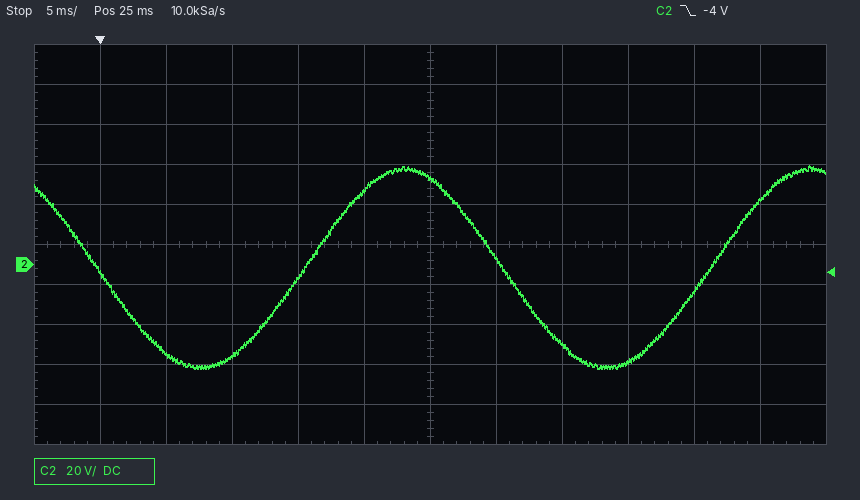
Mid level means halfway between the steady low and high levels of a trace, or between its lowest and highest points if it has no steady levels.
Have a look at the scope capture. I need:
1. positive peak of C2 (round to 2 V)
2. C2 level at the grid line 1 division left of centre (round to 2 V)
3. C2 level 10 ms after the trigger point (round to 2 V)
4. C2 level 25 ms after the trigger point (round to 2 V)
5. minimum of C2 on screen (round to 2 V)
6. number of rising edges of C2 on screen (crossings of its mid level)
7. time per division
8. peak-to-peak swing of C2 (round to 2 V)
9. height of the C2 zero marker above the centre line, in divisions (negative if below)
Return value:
50 V
36 V
-46 V
44 V
-52 V
2
5 ms
102 V
-0.5 div
